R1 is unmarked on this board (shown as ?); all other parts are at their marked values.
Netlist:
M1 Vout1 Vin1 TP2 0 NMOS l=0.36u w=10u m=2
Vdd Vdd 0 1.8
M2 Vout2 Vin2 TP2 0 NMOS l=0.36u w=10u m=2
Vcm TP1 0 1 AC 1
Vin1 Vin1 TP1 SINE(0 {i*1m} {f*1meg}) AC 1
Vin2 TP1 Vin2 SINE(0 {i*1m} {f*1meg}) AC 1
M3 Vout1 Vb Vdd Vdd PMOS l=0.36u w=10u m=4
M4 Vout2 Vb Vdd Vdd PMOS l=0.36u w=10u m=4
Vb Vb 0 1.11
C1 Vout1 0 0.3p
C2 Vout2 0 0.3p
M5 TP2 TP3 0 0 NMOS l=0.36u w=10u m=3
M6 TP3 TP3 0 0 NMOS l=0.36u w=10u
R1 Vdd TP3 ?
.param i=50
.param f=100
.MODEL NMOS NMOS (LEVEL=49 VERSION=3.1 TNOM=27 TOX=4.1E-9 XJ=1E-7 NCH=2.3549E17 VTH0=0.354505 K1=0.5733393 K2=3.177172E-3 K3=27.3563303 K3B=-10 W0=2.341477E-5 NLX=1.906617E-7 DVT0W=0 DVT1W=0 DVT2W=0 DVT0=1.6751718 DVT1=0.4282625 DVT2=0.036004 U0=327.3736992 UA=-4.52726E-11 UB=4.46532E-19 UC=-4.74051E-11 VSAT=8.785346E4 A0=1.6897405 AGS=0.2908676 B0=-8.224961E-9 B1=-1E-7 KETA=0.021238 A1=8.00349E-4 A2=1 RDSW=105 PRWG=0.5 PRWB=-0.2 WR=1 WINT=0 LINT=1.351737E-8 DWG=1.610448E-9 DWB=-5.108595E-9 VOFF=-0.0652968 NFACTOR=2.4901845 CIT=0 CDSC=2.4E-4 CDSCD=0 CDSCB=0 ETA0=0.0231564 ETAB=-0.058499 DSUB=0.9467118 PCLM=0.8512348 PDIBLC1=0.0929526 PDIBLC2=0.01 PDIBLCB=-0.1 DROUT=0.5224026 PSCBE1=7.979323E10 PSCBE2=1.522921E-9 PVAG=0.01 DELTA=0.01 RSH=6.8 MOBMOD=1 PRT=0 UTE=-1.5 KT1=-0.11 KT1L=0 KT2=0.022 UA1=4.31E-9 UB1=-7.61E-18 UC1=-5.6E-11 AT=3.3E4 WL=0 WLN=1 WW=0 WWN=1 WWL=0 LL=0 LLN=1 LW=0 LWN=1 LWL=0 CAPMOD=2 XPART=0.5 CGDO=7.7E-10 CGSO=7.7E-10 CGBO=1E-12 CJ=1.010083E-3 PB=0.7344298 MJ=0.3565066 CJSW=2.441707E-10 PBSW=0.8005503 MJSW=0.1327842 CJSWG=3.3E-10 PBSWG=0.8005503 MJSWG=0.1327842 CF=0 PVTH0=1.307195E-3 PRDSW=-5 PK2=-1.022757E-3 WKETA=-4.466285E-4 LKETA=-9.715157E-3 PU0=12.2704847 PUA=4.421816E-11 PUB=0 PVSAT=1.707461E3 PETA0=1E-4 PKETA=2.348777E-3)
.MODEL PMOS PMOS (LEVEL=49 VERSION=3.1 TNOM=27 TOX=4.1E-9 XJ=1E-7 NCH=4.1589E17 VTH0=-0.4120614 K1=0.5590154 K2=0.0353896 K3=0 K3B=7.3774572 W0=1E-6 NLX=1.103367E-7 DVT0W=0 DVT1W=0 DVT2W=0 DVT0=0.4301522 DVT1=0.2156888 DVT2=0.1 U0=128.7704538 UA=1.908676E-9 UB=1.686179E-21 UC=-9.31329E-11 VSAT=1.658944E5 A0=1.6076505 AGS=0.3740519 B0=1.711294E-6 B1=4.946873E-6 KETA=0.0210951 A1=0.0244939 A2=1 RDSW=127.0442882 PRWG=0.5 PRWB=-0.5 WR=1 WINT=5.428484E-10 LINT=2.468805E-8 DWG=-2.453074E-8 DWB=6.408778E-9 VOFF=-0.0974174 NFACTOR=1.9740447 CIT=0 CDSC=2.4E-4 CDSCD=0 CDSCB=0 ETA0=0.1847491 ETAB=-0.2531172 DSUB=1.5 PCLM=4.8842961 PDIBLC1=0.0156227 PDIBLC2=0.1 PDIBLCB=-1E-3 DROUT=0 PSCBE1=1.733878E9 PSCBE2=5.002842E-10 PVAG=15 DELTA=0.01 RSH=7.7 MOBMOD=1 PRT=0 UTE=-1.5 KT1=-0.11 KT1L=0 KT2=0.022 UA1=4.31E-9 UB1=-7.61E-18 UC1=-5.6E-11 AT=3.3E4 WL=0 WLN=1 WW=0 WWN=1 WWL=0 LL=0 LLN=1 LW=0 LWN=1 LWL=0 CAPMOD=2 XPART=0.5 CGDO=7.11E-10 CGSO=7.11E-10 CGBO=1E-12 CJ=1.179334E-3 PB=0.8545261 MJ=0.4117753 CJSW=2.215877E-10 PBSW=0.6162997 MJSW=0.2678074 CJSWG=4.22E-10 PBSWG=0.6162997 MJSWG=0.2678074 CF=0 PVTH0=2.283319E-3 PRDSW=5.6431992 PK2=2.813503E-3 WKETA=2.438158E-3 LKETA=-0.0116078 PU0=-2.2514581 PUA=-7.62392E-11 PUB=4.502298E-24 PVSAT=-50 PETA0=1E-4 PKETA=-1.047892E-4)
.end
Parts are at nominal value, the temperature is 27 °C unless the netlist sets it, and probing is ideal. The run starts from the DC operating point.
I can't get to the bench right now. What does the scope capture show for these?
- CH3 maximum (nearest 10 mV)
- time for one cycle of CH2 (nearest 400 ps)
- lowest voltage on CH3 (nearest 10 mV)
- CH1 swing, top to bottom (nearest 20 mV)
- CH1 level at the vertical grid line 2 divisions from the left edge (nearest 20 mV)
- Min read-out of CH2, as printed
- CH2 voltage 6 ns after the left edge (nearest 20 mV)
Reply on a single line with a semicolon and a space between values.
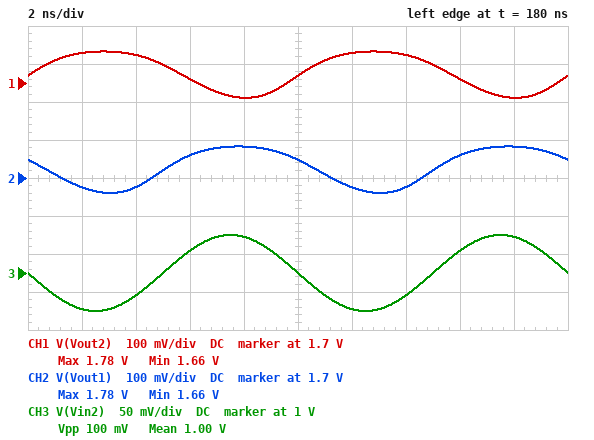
1.05 V; 10.0 ns; 950 mV; 120 mV; 1.78 V; 1.66 V; 1.76 V
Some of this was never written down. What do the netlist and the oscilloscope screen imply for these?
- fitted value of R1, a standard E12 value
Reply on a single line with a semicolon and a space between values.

18 kΩ
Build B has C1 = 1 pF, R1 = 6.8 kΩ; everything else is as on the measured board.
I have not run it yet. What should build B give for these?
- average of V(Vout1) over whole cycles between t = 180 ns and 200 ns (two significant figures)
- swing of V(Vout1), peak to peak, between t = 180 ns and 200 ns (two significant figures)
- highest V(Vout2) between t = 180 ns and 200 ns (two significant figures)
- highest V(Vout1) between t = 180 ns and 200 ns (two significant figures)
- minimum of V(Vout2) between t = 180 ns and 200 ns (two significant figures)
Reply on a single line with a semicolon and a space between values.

200 mV; 14 mV; 220 mV; 210 mV; 190 mV
